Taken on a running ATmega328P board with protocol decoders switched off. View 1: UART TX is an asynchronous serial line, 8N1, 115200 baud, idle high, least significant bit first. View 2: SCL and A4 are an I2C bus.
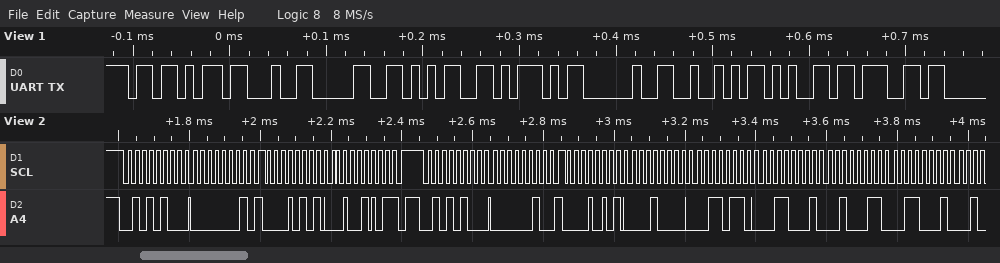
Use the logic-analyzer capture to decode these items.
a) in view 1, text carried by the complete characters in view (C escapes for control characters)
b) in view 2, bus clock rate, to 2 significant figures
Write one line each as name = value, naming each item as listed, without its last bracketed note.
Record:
in view 1, text carried by the complete characters in view = "[#05] Reg"
in view 2, bus clock rate, to 2 significant figures = 50 kHz
